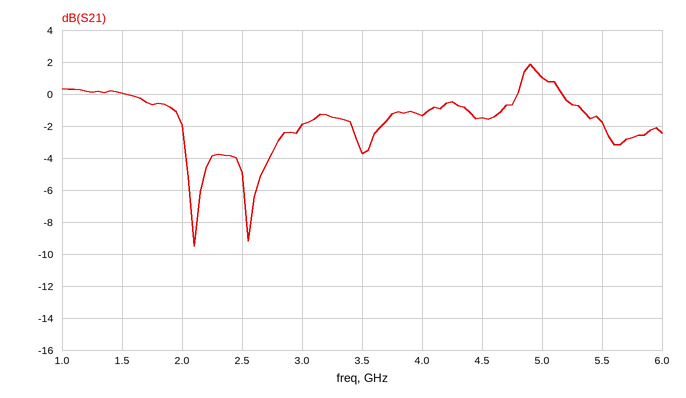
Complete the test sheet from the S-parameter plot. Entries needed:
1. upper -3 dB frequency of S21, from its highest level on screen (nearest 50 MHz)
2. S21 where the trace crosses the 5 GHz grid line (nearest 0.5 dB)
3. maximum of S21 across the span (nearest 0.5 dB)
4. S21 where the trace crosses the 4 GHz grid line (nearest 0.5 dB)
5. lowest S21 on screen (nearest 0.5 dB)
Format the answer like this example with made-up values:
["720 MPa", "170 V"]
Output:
["5.35 GHz", "1.0 dB", "2.0 dB", "-1.5 dB", "-9.5 dB"]
